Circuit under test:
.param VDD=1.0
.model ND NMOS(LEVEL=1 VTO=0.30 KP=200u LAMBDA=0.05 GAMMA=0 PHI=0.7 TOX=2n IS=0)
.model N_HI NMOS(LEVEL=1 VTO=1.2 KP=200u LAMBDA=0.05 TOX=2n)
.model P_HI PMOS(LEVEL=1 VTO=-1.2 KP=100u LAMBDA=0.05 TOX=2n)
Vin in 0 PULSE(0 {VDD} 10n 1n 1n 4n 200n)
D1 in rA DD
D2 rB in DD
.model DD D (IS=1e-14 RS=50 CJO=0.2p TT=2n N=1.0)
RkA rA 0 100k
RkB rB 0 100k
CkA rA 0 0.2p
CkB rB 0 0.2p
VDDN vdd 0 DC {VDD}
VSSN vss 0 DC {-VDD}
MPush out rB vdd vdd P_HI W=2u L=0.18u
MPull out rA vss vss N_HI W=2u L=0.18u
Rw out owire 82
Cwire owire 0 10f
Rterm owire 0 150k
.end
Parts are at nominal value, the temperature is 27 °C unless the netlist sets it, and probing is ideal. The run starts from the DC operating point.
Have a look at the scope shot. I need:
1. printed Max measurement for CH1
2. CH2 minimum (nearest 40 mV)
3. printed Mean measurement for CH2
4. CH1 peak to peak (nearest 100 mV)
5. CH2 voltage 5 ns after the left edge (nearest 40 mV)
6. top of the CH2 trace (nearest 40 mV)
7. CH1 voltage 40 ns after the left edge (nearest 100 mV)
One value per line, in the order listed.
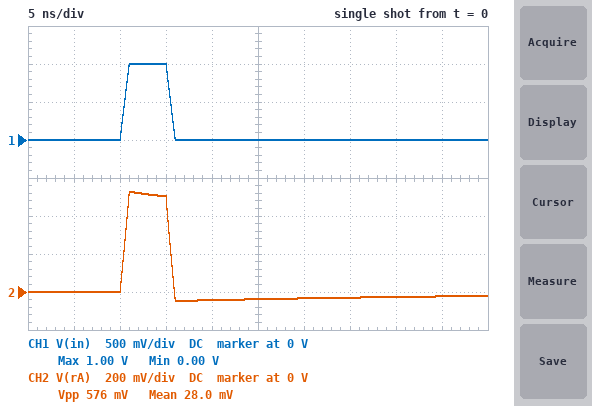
1.00 V
-40 mV
28.0 mV
1.0 V
0 V
520 mV
0 V
